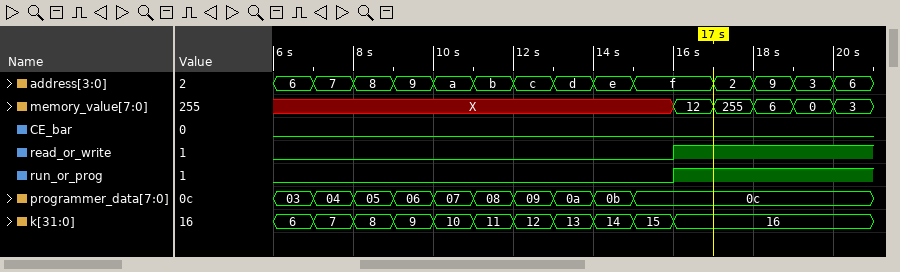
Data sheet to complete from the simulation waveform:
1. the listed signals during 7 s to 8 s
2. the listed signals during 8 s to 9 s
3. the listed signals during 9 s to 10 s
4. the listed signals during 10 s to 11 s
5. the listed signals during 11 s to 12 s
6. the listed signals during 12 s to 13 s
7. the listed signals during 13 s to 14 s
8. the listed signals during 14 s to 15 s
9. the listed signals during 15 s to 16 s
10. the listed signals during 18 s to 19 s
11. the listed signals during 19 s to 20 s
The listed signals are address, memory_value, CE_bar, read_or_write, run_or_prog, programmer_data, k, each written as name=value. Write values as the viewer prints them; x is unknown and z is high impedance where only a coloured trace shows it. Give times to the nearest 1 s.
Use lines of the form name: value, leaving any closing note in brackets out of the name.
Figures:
the listed signals during 7 s to 8 s: address=7, memory_value=X, CE_bar=0, read_or_write=0, run_or_prog=0, programmer_data=04, k=7
the listed signals during 8 s to 9 s: address=8, memory_value=X, CE_bar=0, read_or_write=0, run_or_prog=0, programmer_data=05, k=8
the listed signals during 9 s to 10 s: address=9, memory_value=X, CE_bar=0, read_or_write=0, run_or_prog=0, programmer_data=06, k=9
the listed signals during 10 s to 11 s: address=a, memory_value=X, CE_bar=0, read_or_write=0, run_or_prog=0, programmer_data=07, k=10
the listed signals during 11 s to 12 s: address=b, memory_value=X, CE_bar=0, read_or_write=0, run_or_prog=0, programmer_data=08, k=11
the listed signals during 12 s to 13 s: address=c, memory_value=X, CE_bar=0, read_or_write=0, run_or_prog=0, programmer_data=09, k=12
the listed signals during 13 s to 14 s: address=d, memory_value=X, CE_bar=0, read_or_write=0, run_or_prog=0, programmer_data=0a, k=13
the listed signals during 14 s to 15 s: address=e, memory_value=X, CE_bar=0, read_or_write=0, run_or_prog=0, programmer_data=0b, k=14
the listed signals during 15 s to 16 s: address=f, memory_value=X, CE_bar=0, read_or_write=0, run_or_prog=0, programmer_data=0c, k=15
the listed signals during 18 s to 19 s: address=9, memory_value=6, CE_bar=0, read_or_write=1, run_or_prog=1, programmer_data=0c, k=16
the listed signals during 19 s to 20 s: address=3, memory_value=0, CE_bar=0, read_or_write=1, run_or_prog=1, programmer_data=0c, k=16
